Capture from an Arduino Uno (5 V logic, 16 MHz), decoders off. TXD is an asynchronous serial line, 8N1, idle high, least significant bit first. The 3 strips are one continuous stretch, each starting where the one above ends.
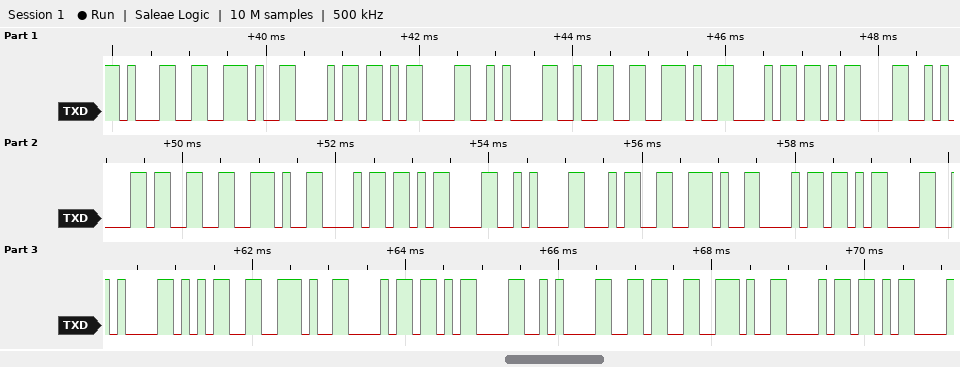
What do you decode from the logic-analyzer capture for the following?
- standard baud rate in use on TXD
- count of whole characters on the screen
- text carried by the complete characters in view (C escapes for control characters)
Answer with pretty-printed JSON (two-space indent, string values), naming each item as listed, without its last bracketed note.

{
  "standard baud rate in use on TXD": "9600 baud",
  "count of whole characters on the screen": "29",
  "text carried by the complete characters in view": "\"1.h\\r\\n2.h\\r\\n3.h\\r\\n4.h\\r\\n5.h\\r\\n6.h\\r\""
}
